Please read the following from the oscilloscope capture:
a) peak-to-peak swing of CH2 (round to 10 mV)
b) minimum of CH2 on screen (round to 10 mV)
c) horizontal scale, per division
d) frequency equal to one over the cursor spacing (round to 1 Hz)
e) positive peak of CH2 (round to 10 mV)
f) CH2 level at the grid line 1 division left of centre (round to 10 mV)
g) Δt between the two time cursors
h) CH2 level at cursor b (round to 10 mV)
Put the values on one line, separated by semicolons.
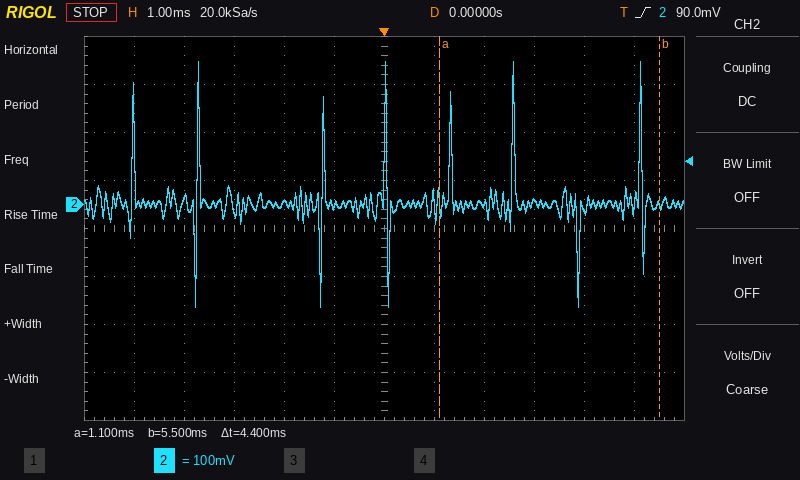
510 mV; -210 mV; 1 ms; 227 Hz; 300 mV; 0 mV; 4.4 ms; 0 mV
